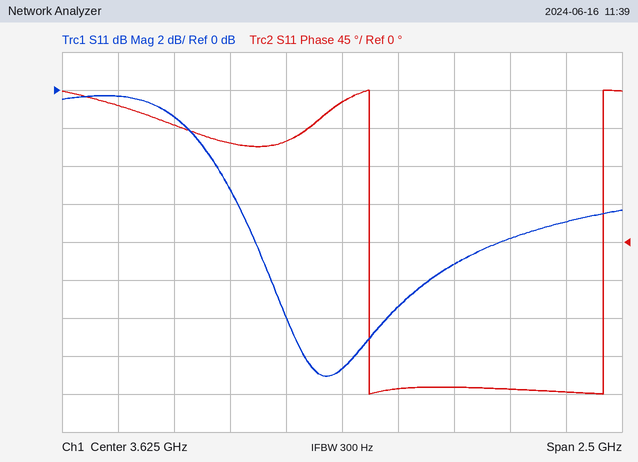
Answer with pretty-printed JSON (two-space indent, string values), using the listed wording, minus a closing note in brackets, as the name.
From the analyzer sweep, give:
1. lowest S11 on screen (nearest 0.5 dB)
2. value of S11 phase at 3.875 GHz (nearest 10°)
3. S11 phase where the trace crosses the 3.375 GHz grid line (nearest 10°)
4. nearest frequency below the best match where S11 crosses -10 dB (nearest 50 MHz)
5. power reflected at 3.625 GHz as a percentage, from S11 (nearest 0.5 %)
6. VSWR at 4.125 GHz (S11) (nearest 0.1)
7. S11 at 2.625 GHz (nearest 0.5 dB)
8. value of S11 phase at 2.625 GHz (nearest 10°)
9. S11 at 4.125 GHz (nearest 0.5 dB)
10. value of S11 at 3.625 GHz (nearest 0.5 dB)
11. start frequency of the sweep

{
  "lowest S11 on screen": "-15.0 dB",
  "value of S11 phase at 3.875 GHz": "-170°",
  "S11 phase where the trace crosses the 3.375 GHz grid line": "120°",
  "nearest frequency below the best match where S11 crosses -10 dB": "3.30 GHz",
  "power reflected at 3.625 GHz as a percentage, from S11": "3.5 %",
  "VSWR at 4.125 GHz (S11)": "2.1",
  "S11 at 2.625 GHz": "-0.5 dB",
  "value of S11 phase at 2.625 GHz": "160°",
  "S11 at 4.125 GHz": "-9.0 dB",
  "value of S11 at 3.625 GHz": "-14.5 dB",
  "start frequency of the sweep": "2.375 GHz"
}
